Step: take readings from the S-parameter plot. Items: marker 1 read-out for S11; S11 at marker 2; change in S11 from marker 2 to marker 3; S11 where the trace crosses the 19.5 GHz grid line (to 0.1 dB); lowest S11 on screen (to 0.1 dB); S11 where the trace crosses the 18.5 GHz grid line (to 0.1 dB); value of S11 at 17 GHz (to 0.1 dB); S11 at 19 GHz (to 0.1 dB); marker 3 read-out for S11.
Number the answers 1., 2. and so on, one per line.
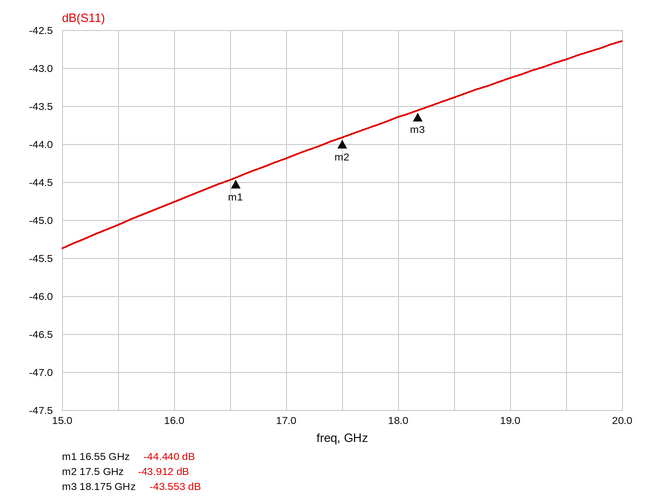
1. -44.440 dB
2. -43.912 dB
3. 0.359 dB
4. -42.9 dB
5. -45.4 dB
6. -43.4 dB
7. -44.2 dB
8. -43.1 dB
9. -43.553 dB
